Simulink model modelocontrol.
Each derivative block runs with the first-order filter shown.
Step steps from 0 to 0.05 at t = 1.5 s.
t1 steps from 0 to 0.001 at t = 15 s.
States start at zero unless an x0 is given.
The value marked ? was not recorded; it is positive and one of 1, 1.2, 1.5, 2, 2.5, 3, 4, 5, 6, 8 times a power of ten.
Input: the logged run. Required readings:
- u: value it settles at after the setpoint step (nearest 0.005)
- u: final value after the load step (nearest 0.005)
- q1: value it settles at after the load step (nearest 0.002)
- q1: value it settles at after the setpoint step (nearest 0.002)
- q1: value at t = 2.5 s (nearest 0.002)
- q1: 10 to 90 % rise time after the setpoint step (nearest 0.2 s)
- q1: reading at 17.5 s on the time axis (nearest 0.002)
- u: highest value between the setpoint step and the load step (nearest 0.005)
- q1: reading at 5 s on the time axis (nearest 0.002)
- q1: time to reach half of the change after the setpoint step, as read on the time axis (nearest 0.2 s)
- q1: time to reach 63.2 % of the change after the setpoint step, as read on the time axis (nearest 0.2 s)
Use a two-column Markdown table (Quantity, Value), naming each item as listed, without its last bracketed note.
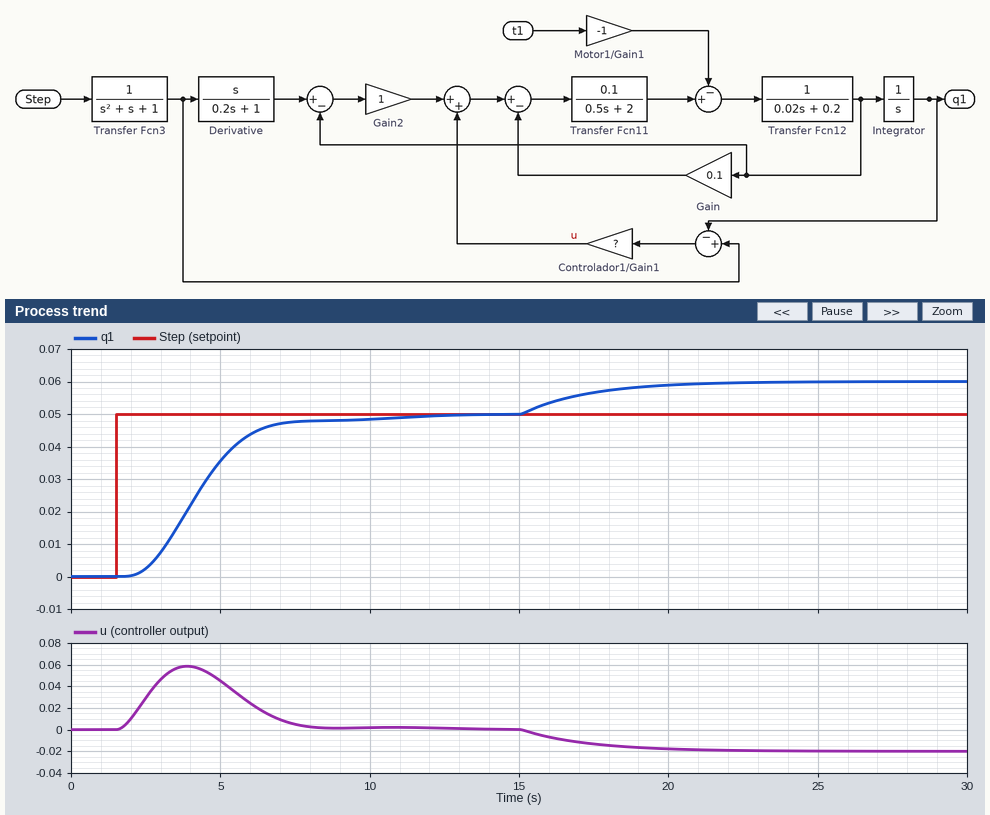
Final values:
| Quantity | Value |
|---|---|
| u: value it settles at after the setpoint step | 0.000 |
| u: final value after the load step | -0.020 |
| q1: value it settles at after the load step | 0.060 |
| q1: value it settles at after the setpoint step | 0.050 |
| q1: value at t = 2.5 s | 0.002 |
| q1: 10 to 90 % rise time after the setpoint step | 3.4 s |
| q1: reading at 17.5 s on the time axis | 0.056 |
| u: highest value between the setpoint step and the load step | 0.060 |
| q1: reading at 5 s on the time axis | 0.036 |
| q1: time to reach half of the change after the setpoint step, as read on the time axis | 4.2 s |
| q1: time to reach 63.2 % of the change after the setpoint step, as read on the time axis | 4.6 s |
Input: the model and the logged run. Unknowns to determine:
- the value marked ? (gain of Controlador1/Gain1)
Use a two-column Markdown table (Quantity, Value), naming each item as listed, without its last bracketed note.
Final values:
| Quantity | Value |
|---|---|
| the value marked ? | 2 |
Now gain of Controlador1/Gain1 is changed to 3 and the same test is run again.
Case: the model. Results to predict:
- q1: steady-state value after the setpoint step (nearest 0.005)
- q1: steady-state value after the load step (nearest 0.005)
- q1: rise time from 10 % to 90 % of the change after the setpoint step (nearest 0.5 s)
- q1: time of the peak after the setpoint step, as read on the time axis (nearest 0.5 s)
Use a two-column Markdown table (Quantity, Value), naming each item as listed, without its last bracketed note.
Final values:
| Quantity | Value |
|---|---|
| q1: steady-state value after the setpoint step | 0.050 |
| q1: steady-state value after the load step | 0.055 |
| q1: rise time from 10 % to 90 % of the change after the setpoint step | 2.5 s |
| q1: time of the peak after the setpoint step, as read on the time axis | 7.0 s |
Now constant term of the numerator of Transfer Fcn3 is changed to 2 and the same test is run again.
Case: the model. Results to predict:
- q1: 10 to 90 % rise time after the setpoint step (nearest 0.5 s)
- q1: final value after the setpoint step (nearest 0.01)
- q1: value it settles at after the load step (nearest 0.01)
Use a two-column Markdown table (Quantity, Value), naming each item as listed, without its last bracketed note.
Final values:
| Quantity | Value |
|---|---|
| q1: 10 to 90 % rise time after the setpoint step | 3.5 s |
| q1: final value after the setpoint step | 0.10 |
| q1: value it settles at after the load step | 0.11 |
